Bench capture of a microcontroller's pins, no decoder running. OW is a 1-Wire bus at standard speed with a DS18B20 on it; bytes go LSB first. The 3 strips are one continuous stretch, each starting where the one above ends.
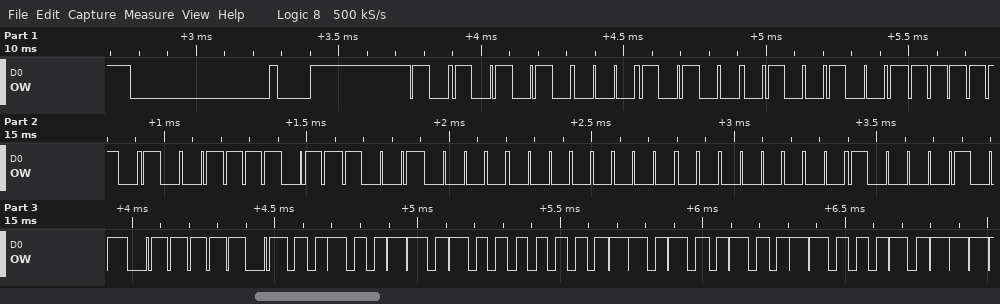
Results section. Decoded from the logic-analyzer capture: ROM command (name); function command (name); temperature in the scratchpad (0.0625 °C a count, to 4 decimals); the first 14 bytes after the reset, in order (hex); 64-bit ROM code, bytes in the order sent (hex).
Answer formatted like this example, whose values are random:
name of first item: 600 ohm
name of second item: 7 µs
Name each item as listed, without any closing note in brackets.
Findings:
ROM command: Match ROM
function command: Read Scratchpad
temperature in the scratchpad: 22.2500 °C
the first 14 bytes after the reset, in order: 55 28 92 5F DE 09 00 00 A1 BE 64 01 4B 46
64-bit ROM code, bytes in the order sent: 28 92 5F DE 09 00 00 A1
